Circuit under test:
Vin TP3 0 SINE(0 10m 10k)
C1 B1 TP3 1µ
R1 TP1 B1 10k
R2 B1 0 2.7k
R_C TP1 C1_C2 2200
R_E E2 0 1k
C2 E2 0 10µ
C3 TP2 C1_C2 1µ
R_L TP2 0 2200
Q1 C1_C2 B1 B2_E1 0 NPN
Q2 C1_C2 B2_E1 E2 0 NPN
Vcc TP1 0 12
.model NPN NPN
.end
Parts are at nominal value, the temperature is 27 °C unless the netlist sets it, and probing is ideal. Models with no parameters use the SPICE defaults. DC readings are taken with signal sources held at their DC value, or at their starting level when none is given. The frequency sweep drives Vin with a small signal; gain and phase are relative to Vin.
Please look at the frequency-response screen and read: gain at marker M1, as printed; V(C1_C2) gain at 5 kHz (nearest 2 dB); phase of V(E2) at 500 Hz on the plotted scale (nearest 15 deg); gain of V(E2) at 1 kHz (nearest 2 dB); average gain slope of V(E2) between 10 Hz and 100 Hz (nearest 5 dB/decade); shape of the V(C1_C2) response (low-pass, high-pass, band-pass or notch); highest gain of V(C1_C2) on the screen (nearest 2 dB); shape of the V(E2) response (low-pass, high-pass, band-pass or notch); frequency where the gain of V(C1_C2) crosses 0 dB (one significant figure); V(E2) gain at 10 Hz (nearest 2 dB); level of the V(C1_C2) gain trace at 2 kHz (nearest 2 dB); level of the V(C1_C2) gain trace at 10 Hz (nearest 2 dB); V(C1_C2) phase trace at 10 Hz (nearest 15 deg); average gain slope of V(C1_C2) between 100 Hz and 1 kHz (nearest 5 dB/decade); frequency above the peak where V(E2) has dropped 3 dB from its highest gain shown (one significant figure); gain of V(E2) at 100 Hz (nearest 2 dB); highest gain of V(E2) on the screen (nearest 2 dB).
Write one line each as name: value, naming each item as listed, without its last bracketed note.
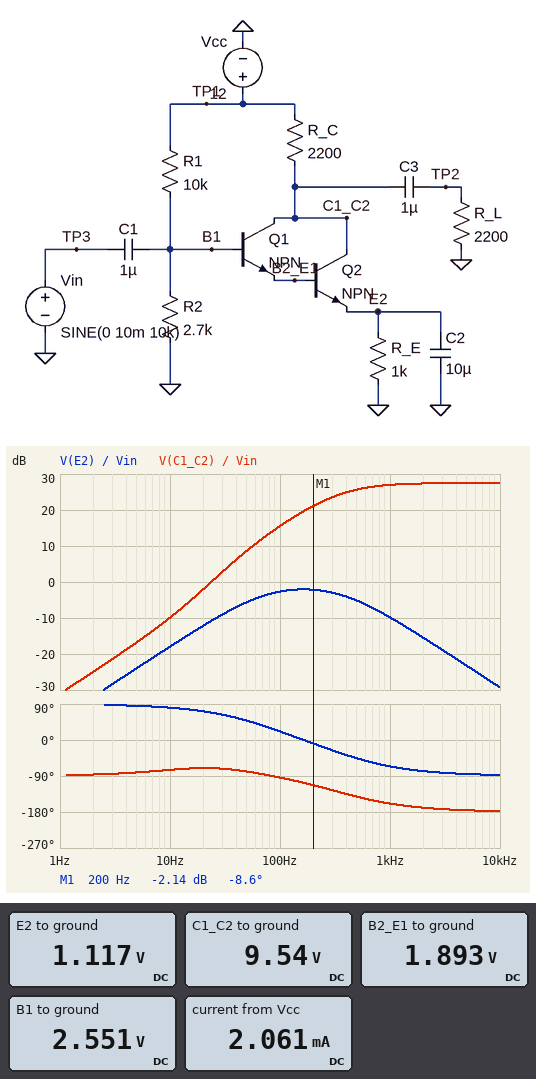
gain at marker M1, as printed: -2.14 dB
V(C1_C2) gain at 5 kHz: 28 dB
phase of V(E2) at 500 Hz on the plotted scale: -45 deg
gain of V(E2) at 1 kHz: -10 dB
average gain slope of V(E2) between 10 Hz and 100 Hz: 15 dB/decade
shape of the V(C1_C2) response: high-pass
highest gain of V(C1_C2) on the screen: 28 dB
shape of the V(E2) response: band-pass
frequency where the gain of V(C1_C2) crosses 0 dB: 20 Hz
V(E2) gain at 10 Hz: -18 dB
level of the V(C1_C2) gain trace at 2 kHz: 28 dB
level of the V(C1_C2) gain trace at 10 Hz: -10 dB
V(C1_C2) phase trace at 10 Hz: -75 deg
average gain slope of V(C1_C2) between 100 Hz and 1 kHz: 10 dB/decade
frequency above the peak where V(E2) has dropped 3 dB from its highest gain shown: 500 Hz
gain of V(E2) at 100 Hz: -2 dB
highest gain of V(E2) on the screen: -2 dB
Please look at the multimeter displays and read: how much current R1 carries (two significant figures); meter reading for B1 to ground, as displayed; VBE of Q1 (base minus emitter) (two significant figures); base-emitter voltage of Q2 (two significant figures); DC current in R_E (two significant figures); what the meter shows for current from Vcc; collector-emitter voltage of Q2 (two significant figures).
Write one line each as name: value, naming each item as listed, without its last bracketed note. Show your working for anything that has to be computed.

how much current R1 carries: (12 V - 2.551 V) / 10 kΩ = 940 µA
meter reading for B1 to ground, as displayed: 2.551 V
VBE of Q1 (base minus emitter): 2.551 V - 1.893 V = 660 mV
base-emitter voltage of Q2: 1.893 V - 1.117 V = 780 mV
DC current in R_E: (1.117 V) / 1 kΩ = 1.1 mA
what the meter shows for current from Vcc: 2.061 mA
collector-emitter voltage of Q2: 9.54 V - 1.117 V = 8.4 V
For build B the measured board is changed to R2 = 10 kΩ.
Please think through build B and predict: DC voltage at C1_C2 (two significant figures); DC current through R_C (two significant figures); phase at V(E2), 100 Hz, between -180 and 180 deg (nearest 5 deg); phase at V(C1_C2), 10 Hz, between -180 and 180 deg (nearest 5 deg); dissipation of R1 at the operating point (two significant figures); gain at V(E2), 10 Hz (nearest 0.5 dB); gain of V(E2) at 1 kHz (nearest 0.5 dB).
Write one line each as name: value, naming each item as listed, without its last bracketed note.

DC voltage at C1_C2: 4.4 V
DC current through R_C: 3.4 mA
phase at V(E2), 100 Hz, between -180 and 180 deg: 10 deg
phase at V(C1_C2), 10 Hz, between -180 and 180 deg: 65 deg
dissipation of R1 at the operating point: 4.7 mW
gain at V(E2), 10 Hz: -29.5 dB
gain of V(E2) at 1 kHz: -23.0 dB
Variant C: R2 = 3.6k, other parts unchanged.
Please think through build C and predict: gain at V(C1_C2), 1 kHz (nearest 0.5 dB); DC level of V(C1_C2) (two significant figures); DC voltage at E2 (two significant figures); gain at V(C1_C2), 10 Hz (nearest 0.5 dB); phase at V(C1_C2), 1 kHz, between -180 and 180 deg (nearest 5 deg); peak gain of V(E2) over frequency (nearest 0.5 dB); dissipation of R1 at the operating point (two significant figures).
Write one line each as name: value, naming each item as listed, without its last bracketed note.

gain at V(C1_C2), 1 kHz: 30.0 dB
DC level of V(C1_C2): 8.2 V
DC voltage at E2: 1.7 V
gain at V(C1_C2), 10 Hz: -8.0 dB
phase at V(C1_C2), 1 kHz, between -180 and 180 deg: -150 deg
peak gain of V(E2) over frequency: -1.0 dB
dissipation of R1 at the operating point: 7.8 mW
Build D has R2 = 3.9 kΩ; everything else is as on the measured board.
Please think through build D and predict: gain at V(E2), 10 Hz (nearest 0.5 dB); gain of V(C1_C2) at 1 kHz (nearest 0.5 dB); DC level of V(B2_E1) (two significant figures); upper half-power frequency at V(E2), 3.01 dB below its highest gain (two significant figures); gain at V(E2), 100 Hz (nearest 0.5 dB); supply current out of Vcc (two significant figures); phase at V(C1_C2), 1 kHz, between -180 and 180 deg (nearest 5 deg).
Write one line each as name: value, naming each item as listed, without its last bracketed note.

gain at V(E2), 10 Hz: -15.5 dB
gain of V(C1_C2) at 1 kHz: 31.0 dB
DC level of V(B2_E1): 2.7 V
upper half-power frequency at V(E2), 3.01 dB below its highest gain: 710 Hz
gain at V(E2), 100 Hz: -1.5 dB
supply current out of Vcc: 2.8 mA
phase at V(C1_C2), 1 kHz, between -180 and 180 deg: -150 deg
